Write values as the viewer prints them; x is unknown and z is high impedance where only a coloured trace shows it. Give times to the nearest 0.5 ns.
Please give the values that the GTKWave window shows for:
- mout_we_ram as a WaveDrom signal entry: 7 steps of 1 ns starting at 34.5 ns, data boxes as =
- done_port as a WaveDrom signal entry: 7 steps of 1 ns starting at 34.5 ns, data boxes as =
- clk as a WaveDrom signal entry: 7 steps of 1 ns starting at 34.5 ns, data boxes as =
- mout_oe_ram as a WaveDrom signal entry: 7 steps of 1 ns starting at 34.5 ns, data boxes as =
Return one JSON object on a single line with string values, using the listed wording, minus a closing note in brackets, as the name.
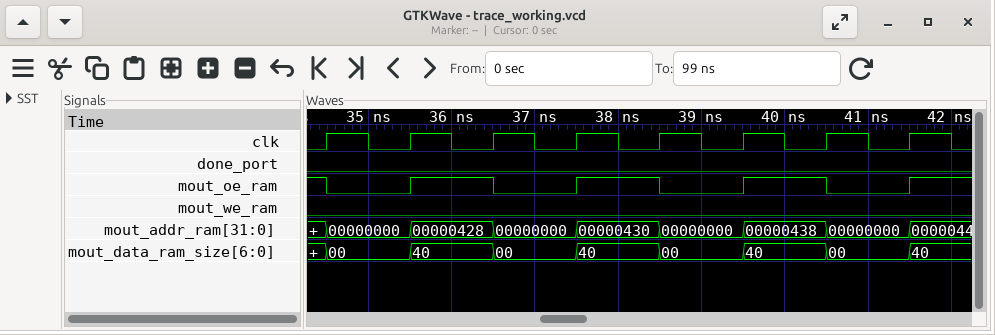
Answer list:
{"mout_we_ram as a WaveDrom signal entry: 7 steps of 1 ns starting at 34.5 ns, data boxes as =": "{name: 'mout_we_ram', wave: '0......'}", "done_port as a WaveDrom signal entry: 7 steps of 1 ns starting at 34.5 ns, data boxes as =": "{name: 'done_port', wave: '0......'}", "clk as a WaveDrom signal entry: 7 steps of 1 ns starting at 34.5 ns, data boxes as =": "{name: 'clk', wave: 'p......'}", "mout_oe_ram as a WaveDrom signal entry: 7 steps of 1 ns starting at 34.5 ns, data boxes as =": "{name: 'mout_oe_ram', wave: '0101010'}"}
